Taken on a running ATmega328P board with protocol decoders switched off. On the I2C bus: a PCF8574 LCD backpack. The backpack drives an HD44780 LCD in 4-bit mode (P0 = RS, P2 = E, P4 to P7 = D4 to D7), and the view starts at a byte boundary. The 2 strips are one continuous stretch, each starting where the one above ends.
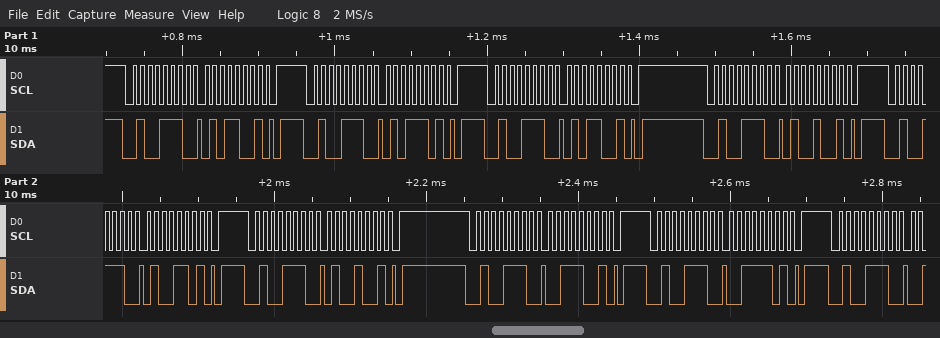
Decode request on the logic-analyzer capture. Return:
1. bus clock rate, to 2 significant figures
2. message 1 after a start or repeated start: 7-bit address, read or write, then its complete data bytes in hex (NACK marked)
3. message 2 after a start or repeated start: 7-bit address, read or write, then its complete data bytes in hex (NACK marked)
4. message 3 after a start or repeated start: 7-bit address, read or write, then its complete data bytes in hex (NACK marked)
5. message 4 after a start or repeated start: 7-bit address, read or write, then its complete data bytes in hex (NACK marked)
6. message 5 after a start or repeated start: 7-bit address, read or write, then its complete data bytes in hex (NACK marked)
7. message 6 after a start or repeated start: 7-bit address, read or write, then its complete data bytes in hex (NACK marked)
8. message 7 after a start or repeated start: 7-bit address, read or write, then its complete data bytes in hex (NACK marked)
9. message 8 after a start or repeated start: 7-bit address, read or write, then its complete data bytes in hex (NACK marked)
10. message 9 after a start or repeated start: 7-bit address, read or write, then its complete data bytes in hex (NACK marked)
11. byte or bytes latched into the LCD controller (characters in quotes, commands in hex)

100 kHz
0x27 write: 59
0x27 write: 5D
0x27 write: 59
0x27 write: 49
0x27 write: 4D
0x27 write: 49
0x27 write: 39
0x27 write: 3D
0x27 write
'T'
